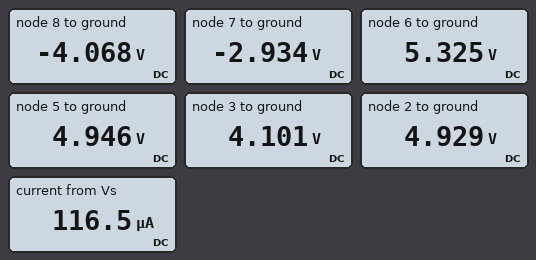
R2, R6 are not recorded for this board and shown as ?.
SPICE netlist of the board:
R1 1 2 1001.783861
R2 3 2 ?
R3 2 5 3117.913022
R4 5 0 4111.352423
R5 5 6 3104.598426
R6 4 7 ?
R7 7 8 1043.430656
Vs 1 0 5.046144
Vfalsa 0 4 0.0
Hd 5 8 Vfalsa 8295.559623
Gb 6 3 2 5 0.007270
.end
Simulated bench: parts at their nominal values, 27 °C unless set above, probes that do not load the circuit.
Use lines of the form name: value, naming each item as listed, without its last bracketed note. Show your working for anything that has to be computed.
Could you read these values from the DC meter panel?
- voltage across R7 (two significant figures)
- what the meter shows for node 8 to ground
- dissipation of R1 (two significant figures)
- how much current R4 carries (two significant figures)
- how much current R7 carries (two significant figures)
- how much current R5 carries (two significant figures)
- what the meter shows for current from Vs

voltage across R7: -2.934 V - (-4.068 V) = 1.1 V
what the meter shows for node 8 to ground: -4.068 V
dissipation of R1: (5.046 V - 4.929 V)^2 / 1.002 kΩ = 14 µW
how much current R4 carries: (4.946 V) / 4.111 kΩ = 1.2 mA
how much current R7 carries: (-2.934 V - (-4.068 V)) / 1.043 kΩ = 1.1 mA
how much current R5 carries: (5.325 V - 4.946 V) / 3.105 kΩ = 120 µA
what the meter shows for current from Vs: 116.5 µA
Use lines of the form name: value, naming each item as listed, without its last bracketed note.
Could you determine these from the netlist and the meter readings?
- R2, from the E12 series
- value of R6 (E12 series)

R2, from the E12 series: 6.8 kΩ
value of R6: 2.7 kΩ
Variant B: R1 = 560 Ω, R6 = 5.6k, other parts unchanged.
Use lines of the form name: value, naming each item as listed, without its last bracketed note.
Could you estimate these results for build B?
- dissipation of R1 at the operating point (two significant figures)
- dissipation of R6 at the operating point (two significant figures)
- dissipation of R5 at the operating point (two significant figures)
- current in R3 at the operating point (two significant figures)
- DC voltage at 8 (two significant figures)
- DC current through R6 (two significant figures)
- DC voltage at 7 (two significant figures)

dissipation of R1 at the operating point: 2.6 mW
dissipation of R6 at the operating point: 72 mW
dissipation of R5 at the operating point: 16 mW
current in R3 at the operating point: 99 µA
DC voltage at 8: -24 V
DC current through R6: 3.6 mA
DC voltage at 7: -20 V
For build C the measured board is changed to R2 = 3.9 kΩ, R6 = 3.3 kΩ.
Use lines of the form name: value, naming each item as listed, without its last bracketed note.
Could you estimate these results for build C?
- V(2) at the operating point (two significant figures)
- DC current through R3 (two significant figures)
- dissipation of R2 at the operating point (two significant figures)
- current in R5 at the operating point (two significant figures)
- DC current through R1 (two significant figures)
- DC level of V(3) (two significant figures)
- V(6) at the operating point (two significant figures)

V(2) at the operating point: 5.1 V
DC current through R3: 2.3 µA
dissipation of R2 at the operating point: 11 µW
current in R5 at the operating point: 52 µA
DC current through R1: 50 µA
DC level of V(3): 5.3 V
V(6) at the operating point: 4.9 V
